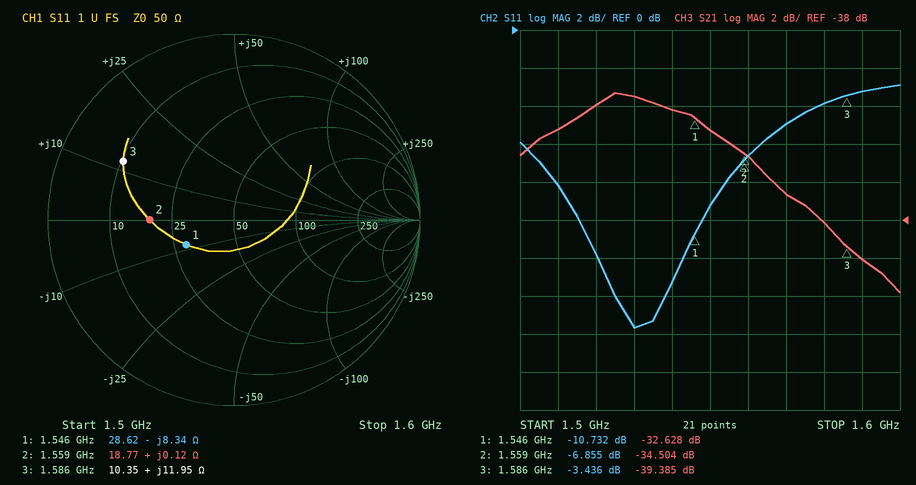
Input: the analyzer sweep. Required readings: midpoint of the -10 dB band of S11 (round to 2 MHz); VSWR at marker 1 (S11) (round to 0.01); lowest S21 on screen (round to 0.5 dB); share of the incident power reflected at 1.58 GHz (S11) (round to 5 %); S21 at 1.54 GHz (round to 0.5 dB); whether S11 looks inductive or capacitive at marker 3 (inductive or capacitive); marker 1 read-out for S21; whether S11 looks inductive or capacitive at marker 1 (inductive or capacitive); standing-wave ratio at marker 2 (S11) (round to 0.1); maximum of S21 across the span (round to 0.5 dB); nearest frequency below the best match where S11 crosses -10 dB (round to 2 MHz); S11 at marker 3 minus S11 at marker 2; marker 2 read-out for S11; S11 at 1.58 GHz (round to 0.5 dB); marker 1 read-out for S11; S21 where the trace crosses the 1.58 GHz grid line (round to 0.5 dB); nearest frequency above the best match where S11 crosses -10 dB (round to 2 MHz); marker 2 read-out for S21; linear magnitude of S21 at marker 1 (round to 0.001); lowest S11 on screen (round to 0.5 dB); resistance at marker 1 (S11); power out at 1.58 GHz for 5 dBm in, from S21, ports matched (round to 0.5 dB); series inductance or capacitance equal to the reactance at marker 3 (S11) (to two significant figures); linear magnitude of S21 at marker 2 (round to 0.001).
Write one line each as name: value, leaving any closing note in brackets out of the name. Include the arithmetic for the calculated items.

midpoint of the -10 dB band of S11: 1.532 GHz
VSWR at marker 1 (S11): 1.82
lowest S21 on screen: -42.0 dB
share of the incident power reflected at 1.58 GHz (S11): 10^(-4/10) ≈ 40 %
S21 at 1.54 GHz: -32.0 dB
whether S11 looks inductive or capacitive at marker 3: inductive
marker 1 read-out for S21: -32.628 dB
whether S11 looks inductive or capacitive at marker 1: capacitive
standing-wave ratio at marker 2 (S11): 2.7
maximum of S21 across the span: -31.5 dB
nearest frequency below the best match where S11 crosses -10 dB: 1.516 GHz
S11 at marker 3 minus S11 at marker 2: -3.436 − (-6.855) = 3.419 dB
marker 2 read-out for S11: -6.855 dB
S11 at 1.58 GHz: -4.0 dB
marker 1 read-out for S11: -10.732 dB
S21 where the trace crosses the 1.58 GHz grid line: -38.0 dB
nearest frequency above the best match where S11 crosses -10 dB: 1.548 GHz
marker 2 read-out for S21: -34.504 dB
linear magnitude of S21 at marker 1: 10^(-32.628/20) ≈ 0.023
lowest S11 on screen: -15.5 dB
resistance at marker 1: 28.62 Ω
power out at 1.58 GHz for 5 dBm in, from S21, ports matched: 5 dBm + (-38.0 dB) = -33.0 dBm
series inductance or capacitance equal to the reactance at marker 3 (S11): L = 11.95 Ω/(2π × 1.586 GHz) ≈ 1.2 nH
linear magnitude of S21 at marker 2: 10^(-34.504/20) ≈ 0.019
